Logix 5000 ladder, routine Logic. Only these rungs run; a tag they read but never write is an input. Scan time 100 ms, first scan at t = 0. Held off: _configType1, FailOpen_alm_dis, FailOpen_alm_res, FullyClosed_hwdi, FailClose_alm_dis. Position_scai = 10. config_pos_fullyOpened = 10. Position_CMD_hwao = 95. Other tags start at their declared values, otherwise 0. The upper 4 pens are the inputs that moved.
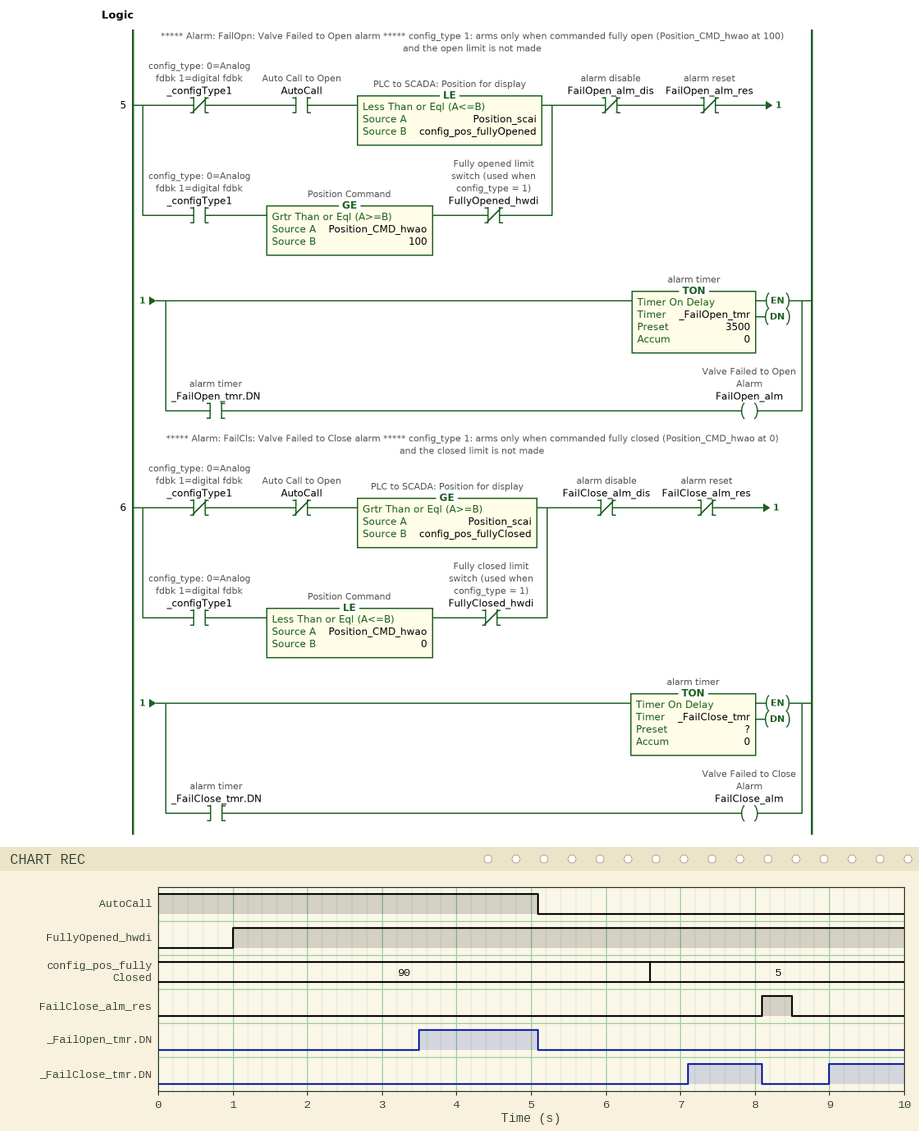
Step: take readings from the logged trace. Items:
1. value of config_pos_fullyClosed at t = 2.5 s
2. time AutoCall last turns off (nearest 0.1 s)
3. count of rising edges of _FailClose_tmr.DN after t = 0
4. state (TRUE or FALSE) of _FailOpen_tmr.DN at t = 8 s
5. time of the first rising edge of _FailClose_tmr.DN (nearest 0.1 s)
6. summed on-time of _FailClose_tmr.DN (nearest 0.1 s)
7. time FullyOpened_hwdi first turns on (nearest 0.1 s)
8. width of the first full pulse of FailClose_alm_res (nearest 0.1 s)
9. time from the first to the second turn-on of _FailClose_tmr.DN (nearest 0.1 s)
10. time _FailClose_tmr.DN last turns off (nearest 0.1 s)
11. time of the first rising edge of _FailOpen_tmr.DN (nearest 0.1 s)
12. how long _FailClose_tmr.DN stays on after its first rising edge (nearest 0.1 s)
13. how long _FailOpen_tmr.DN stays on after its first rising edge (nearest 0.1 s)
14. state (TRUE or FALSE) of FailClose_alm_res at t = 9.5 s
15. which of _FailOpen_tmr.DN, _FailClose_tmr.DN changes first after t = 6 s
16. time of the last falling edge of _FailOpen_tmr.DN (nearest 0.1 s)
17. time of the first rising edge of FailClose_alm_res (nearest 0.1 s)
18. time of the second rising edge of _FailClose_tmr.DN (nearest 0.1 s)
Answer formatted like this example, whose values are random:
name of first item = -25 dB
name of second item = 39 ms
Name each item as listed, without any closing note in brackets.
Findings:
value of config_pos_fullyClosed at t = 2.5 s = 90
time AutoCall last turns off = 5.1 s
count of rising edges of _FailClose_tmr.DN after t = 0 = 2
state (TRUE or FALSE) of _FailOpen_tmr.DN at t = 8 s = FALSE
time of the first rising edge of _FailClose_tmr.DN = 7.1 s
summed on-time of _FailClose_tmr.DN = 2.0 s
time FullyOpened_hwdi first turns on = 1.0 s
width of the first full pulse of FailClose_alm_res = 0.4 s
time from the first to the second turn-on of _FailClose_tmr.DN = 1.9 s
time _FailClose_tmr.DN last turns off = 8.1 s
time of the first rising edge of _FailOpen_tmr.DN = 3.5 s
how long _FailClose_tmr.DN stays on after its first rising edge = 1.0 s
how long _FailOpen_tmr.DN stays on after its first rising edge = 1.6 s
state (TRUE or FALSE) of FailClose_alm_res at t = 9.5 s = FALSE
which of _FailOpen_tmr.DN, _FailClose_tmr.DN changes first after t = 6 s = _FailClose_tmr.DN
time of the last falling edge of _FailOpen_tmr.DN = 5.1 s
time of the first rising edge of FailClose_alm_res = 8.1 s
time of the second rising edge of _FailClose_tmr.DN = 9.0 s
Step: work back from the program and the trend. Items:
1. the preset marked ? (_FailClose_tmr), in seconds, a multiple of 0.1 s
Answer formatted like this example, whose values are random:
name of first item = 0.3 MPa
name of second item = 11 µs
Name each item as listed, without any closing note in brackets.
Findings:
the preset marked ? (_FailClose_tmr), in seconds, a multiple of 0.1 s = 0.5 s
